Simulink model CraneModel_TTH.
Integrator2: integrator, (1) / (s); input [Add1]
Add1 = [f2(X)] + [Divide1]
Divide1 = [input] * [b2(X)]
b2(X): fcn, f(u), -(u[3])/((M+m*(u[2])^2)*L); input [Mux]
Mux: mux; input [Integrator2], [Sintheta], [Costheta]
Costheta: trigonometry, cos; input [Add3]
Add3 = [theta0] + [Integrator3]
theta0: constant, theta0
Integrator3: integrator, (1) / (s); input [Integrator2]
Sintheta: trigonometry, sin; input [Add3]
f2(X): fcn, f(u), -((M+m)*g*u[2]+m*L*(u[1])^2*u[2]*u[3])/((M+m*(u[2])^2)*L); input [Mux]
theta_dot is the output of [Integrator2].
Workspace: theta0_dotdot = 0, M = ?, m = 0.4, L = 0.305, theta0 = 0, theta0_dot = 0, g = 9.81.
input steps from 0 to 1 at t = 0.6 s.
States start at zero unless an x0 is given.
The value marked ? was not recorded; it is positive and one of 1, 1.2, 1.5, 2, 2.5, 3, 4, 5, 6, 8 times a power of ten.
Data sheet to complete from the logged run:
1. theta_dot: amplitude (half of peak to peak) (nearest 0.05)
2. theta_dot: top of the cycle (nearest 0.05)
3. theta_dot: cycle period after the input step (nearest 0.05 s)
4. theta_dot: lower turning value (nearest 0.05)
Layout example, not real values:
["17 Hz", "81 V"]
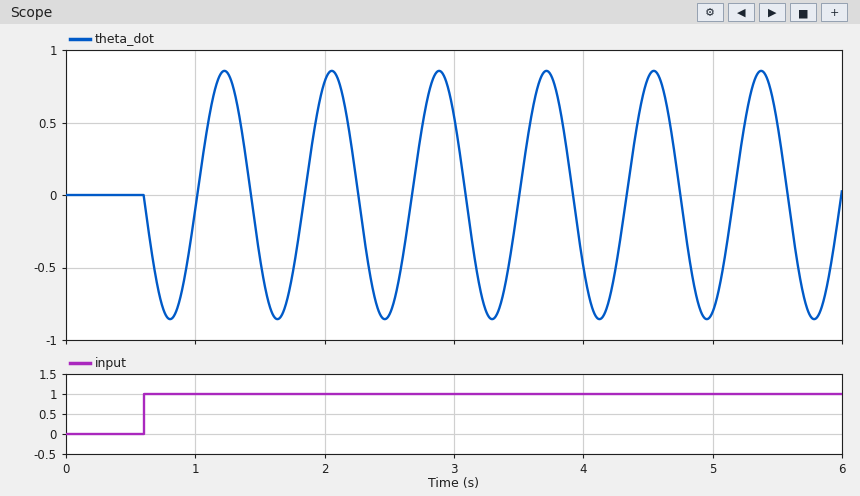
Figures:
["0.85", "0.85", "0.85 s", "-0.85"]
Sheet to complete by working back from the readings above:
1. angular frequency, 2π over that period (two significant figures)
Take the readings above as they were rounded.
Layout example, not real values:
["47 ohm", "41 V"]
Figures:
["7.4 rad/s"]
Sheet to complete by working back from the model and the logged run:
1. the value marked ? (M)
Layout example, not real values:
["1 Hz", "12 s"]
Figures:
["0.5"]
